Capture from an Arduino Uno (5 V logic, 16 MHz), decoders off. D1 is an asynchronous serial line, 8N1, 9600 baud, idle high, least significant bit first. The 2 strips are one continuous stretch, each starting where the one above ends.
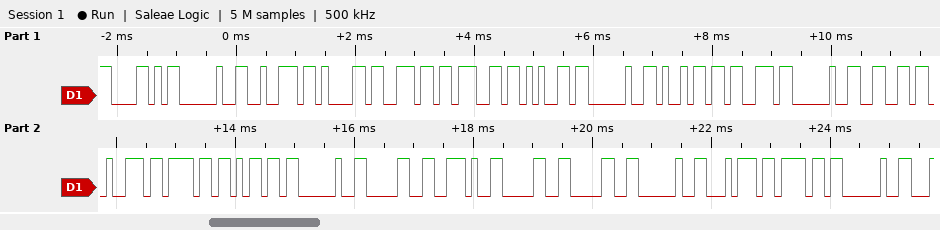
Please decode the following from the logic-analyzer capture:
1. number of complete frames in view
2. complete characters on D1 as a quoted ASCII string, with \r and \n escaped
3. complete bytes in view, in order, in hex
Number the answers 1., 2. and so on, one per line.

1. 24
2. "X range is from 0.00 to "
3. 58 20 72 61 6E 67 65 20 69 73 20 66 72 6F 6D 20 30 2E 30 30 20 74 6F 20
